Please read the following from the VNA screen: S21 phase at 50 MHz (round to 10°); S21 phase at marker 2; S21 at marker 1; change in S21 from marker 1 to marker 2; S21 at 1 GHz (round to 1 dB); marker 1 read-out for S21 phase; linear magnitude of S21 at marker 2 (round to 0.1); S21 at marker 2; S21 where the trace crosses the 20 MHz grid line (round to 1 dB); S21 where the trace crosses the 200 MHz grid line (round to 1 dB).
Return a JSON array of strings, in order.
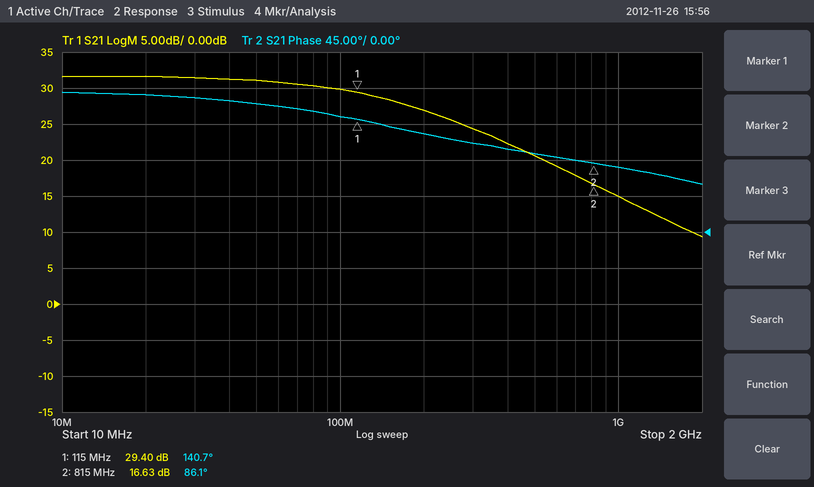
["160°", "86.1°", "29.40 dB", "-12.77 dB", "15 dB", "140.7°", "6.8", "16.63 dB", "32 dB", "27 dB"]
